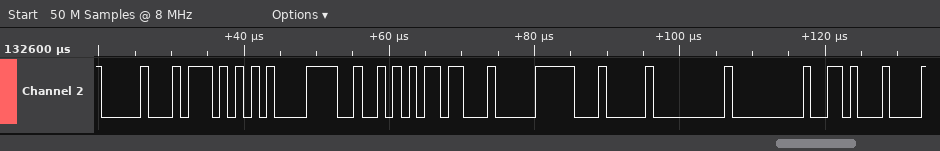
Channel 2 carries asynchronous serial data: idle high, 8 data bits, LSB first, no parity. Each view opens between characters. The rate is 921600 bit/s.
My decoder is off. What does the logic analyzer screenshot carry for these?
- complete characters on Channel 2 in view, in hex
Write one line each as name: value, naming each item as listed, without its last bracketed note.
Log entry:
complete characters on Channel 2 in view, in hex: 10, 57, E1, 52, 1B, F0, 04, 00, 00, 16
